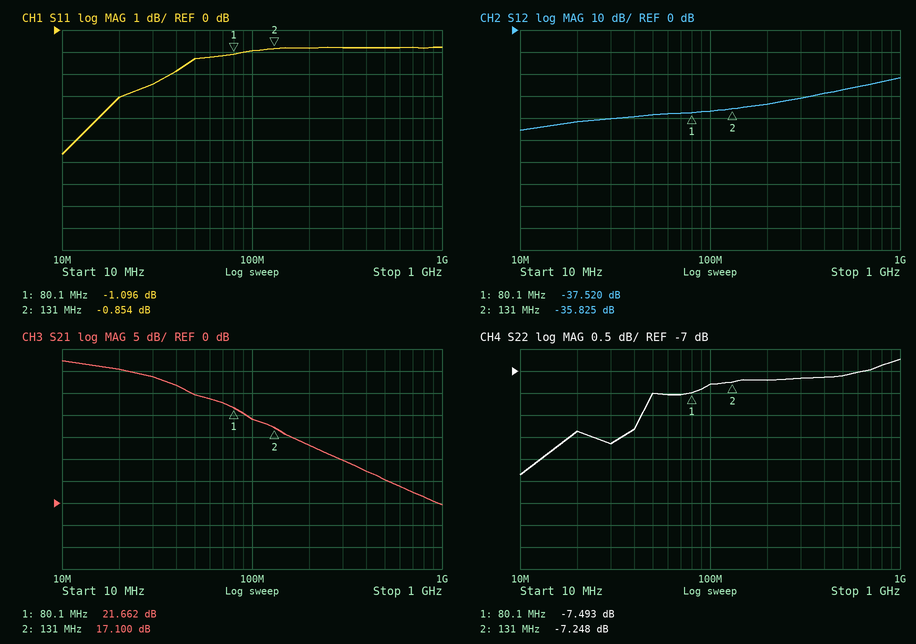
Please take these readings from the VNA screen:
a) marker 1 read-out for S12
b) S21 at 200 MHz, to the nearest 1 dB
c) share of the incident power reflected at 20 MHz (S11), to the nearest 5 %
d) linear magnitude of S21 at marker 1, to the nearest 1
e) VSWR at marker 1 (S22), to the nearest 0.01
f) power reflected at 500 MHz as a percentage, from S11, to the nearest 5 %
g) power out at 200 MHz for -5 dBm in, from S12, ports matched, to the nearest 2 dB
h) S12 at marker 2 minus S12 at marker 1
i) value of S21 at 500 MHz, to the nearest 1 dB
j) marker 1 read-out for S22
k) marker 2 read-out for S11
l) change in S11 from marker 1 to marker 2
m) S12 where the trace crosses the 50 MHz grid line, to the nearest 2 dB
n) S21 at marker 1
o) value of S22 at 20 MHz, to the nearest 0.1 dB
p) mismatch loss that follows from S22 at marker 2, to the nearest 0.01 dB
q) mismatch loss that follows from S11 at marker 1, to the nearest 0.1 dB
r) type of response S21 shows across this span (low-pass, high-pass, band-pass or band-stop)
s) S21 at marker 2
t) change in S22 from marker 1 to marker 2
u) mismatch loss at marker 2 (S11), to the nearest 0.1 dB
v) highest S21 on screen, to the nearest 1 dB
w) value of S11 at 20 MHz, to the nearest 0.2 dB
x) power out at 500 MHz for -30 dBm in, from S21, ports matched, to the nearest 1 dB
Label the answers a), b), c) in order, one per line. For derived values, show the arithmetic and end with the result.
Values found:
a) -37.520 dB
b) 13 dB
c) 10^(-3/10) ≈ 50 %
d) 10^(21.662/20) ≈ 12
e) (1 + 0.4220)/(1 − 0.4220) ≈ 2.46
f) 10^(-0.8/10) ≈ 83.2 %, so 85 % to the nearest 5 %
g) -5 dBm + (-34 dB) = -38 dBm
h) -35.825 − (-37.52) = 1.695 dB
i) 5 dB
j) -7.493 dB
k) -0.854 dB
l) -0.854 − (-1.096) = 0.242 dB
m) -38 dB
n) 21.662 dB
o) -8.4 dB
p) −10 log10(1 − 10^(-7.248/10)) ≈ 0.91 dB
q) −10 log10(1 − 10^(-1.096/10)) ≈ 6.5 dB
r) low-pass
s) 17.100 dB
t) -7.248 − (-7.493) = 0.245 dB
u) −10 log10(1 − 10^(-0.854/10)) ≈ 7.5 dB
v) 32 dB
w) -3.0 dB
x) -30 dBm + (5 dB) = -25 dBm
